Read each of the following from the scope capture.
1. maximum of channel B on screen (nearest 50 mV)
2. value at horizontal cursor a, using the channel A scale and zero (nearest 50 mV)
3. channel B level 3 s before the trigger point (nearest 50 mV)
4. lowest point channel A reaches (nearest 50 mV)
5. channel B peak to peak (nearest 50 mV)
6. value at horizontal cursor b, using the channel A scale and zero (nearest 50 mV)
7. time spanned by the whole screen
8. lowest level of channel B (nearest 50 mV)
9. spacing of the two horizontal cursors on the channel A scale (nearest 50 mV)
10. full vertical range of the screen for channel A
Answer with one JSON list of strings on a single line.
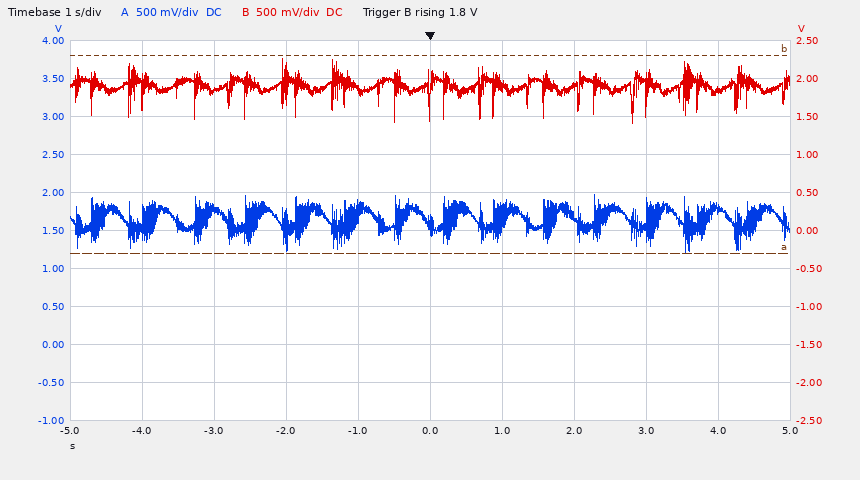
["2.25 V", "1.20 V", "1.85 V", "1.20 V", "850 mV", "3.80 V", "10 s", "1.40 V", "2.60 V", "5 V"]
